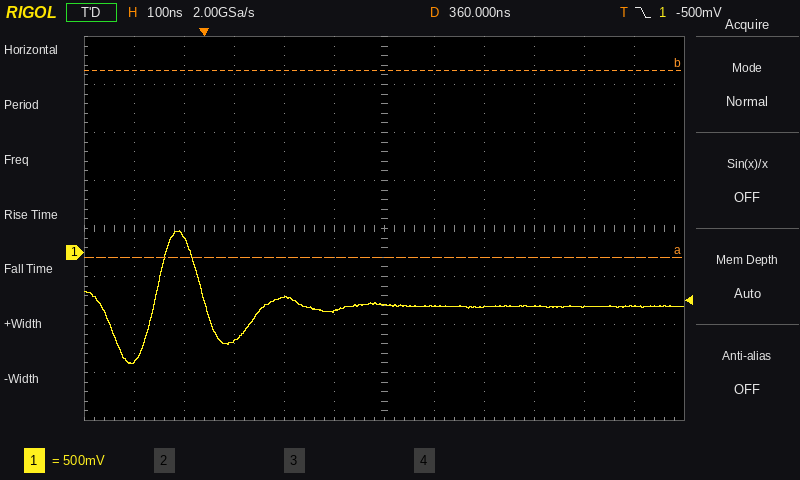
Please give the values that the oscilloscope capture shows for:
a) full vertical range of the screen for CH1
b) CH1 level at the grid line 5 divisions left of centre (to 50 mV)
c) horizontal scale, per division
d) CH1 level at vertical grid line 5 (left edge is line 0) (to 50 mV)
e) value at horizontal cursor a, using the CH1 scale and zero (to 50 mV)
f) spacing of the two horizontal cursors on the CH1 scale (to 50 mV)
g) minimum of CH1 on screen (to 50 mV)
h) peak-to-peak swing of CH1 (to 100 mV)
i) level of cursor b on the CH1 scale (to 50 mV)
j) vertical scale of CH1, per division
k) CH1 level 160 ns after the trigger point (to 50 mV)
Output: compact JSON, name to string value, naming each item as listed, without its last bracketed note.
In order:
{"full vertical range of the screen for CH1": "4 V", "CH1 level at the grid line 5 divisions left of centre": "-1.15 V", "horizontal scale, per division": "100 ns", "CH1 level at vertical grid line 5 (left edge is line 0)": "-600 mV", "value at horizontal cursor a, using the CH1 scale and zero": "-50 mV", "spacing of the two horizontal cursors on the CH1 scale": "1.95 V", "minimum of CH1 on screen": "-1.15 V", "peak-to-peak swing of CH1": "1.40 V", "level of cursor b on the CH1 scale": "1.90 V", "vertical scale of CH1, per division": "500 mV", "CH1 level 160 ns after the trigger point": "-450 mV"}
